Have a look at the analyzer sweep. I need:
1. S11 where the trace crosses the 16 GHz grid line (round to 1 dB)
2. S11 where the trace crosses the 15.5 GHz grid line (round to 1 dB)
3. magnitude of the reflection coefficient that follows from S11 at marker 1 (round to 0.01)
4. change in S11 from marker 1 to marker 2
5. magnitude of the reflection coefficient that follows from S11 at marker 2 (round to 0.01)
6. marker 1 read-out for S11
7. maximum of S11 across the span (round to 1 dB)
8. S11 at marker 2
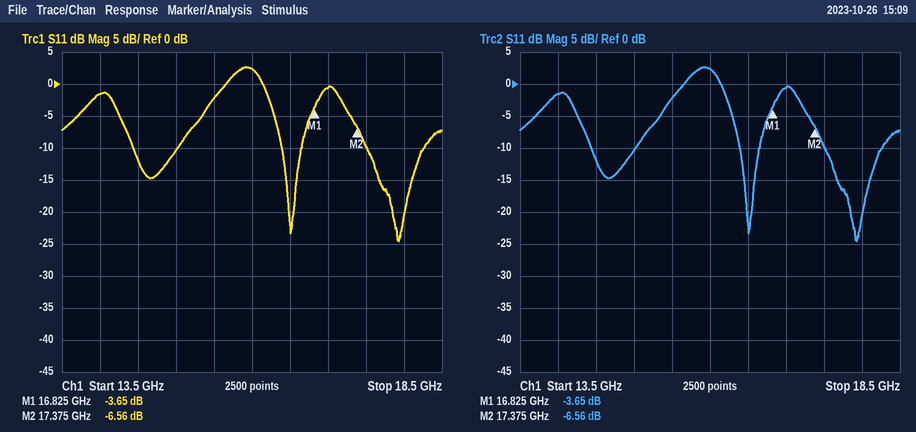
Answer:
2 dB
-2 dB
0.66
-2.91 dB
0.47
-3.65 dB
3 dB
-6.56 dB
